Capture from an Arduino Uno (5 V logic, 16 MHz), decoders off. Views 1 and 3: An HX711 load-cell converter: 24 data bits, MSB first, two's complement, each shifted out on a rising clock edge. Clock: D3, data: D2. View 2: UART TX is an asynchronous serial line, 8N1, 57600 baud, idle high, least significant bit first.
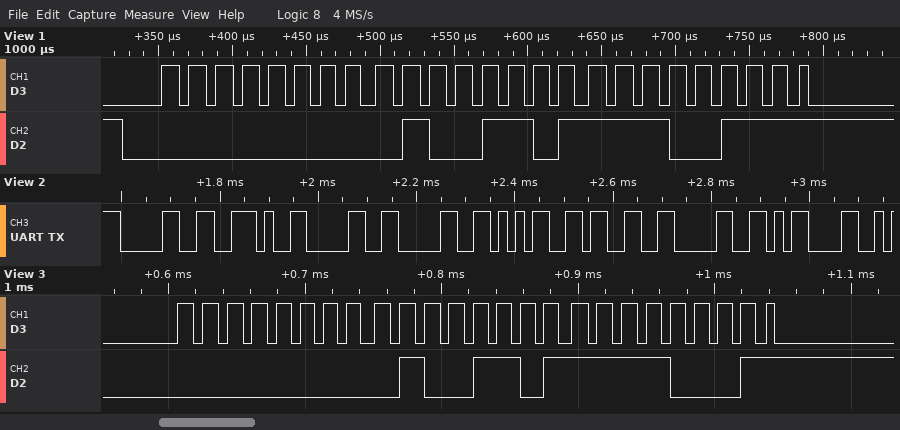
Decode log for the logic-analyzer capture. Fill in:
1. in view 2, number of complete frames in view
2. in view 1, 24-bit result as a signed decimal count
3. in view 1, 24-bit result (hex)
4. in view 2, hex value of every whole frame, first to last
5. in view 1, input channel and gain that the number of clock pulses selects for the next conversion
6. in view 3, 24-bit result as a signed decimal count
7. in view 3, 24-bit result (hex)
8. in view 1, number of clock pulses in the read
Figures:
8
19943
0x004DE7
30 2E 30 30 35 33 30 0D
channel A, gain 128
19953
0x004DF1
25
